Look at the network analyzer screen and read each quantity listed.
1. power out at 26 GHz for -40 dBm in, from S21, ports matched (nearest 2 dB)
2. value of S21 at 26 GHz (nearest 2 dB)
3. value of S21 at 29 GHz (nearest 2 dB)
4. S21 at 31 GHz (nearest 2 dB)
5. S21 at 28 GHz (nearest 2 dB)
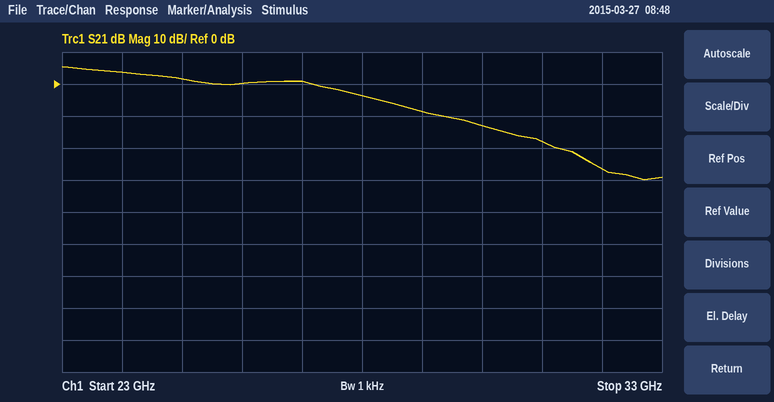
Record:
-40 dBm
0 dB
-8 dB
-18 dB
-4 dB
